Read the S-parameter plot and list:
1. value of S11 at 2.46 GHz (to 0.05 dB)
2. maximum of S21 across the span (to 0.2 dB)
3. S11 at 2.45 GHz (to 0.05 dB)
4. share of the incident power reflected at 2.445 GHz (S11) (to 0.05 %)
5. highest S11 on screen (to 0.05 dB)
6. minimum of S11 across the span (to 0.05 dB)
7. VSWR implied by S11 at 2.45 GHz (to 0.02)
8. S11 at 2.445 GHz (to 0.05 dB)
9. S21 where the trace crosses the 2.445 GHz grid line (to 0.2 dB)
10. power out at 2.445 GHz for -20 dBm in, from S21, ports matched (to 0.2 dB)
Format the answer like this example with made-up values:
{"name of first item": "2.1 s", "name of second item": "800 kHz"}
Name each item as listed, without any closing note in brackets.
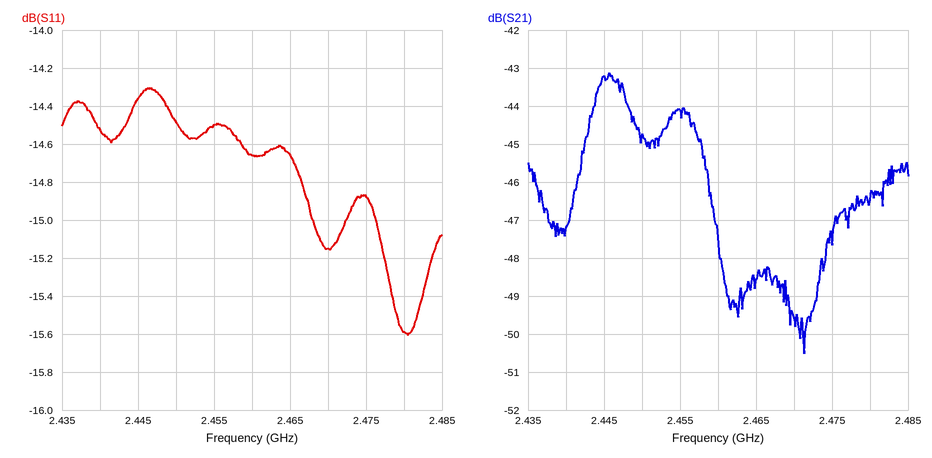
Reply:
{"value of S11 at 2.46 GHz": "-14.65 dB", "maximum of S21 across the span": "-43.2 dB", "S11 at 2.45 GHz": "-14.50 dB", "share of the incident power reflected at 2.445 GHz (S11)": "3.65 %", "highest S11 on screen": "-14.30 dB", "minimum of S11 across the span": "-15.60 dB", "VSWR implied by S11 at 2.45 GHz": "1.46", "S11 at 2.445 GHz": "-14.35 dB", "S21 where the trace crosses the 2.445 GHz grid line": "-43.2 dB", "power out at 2.445 GHz for -20 dBm in, from S21, ports matched": "-63.2 dBm"}
